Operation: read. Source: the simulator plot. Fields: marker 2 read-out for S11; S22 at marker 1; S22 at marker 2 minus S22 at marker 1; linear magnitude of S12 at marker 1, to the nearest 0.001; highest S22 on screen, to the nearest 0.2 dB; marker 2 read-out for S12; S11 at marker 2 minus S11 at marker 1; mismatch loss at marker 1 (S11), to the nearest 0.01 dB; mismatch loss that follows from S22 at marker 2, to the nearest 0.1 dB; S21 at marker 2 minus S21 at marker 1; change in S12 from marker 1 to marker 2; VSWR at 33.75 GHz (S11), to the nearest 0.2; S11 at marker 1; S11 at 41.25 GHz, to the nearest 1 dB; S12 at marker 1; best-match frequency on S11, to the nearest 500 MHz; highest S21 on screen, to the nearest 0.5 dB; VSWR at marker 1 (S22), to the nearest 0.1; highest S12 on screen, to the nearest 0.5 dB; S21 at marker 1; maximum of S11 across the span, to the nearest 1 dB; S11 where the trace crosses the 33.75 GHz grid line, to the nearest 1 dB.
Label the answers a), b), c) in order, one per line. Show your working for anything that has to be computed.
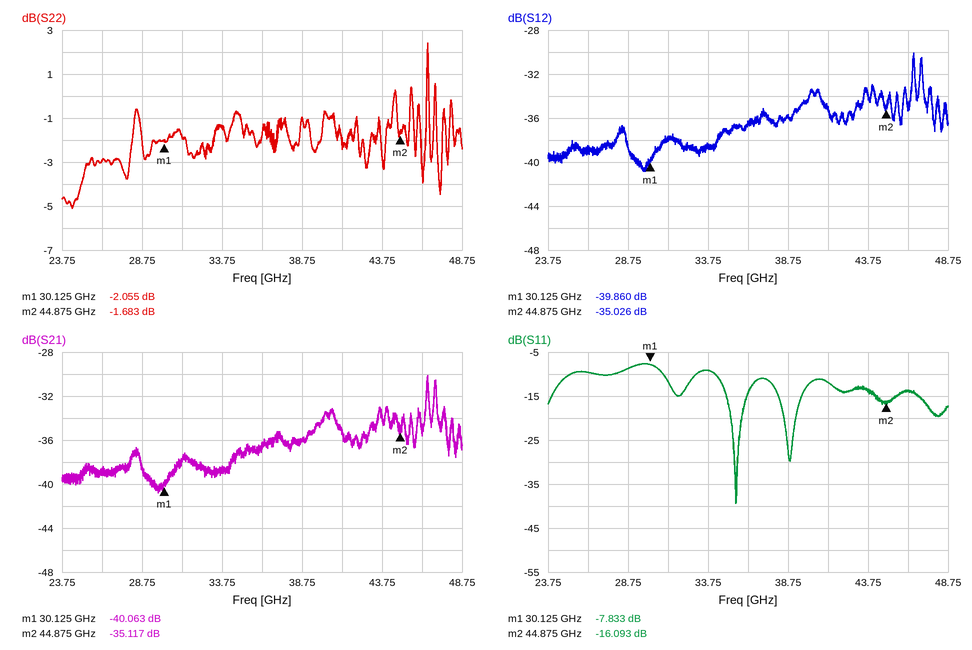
a) -16.093 dB
b) -2.055 dB
c) -1.683 − (-2.055) = 0.372 dB
d) 10^(-39.86/20) ≈ 0.010
e) 2.4 dB
f) -35.026 dB
g) -16.093 − (-7.833) = -8.260 dB
h) −10 log10(1 − 10^(-7.833/10)) ≈ 0.78 dB
i) −10 log10(1 − 10^(-1.683/10)) ≈ 4.9 dB
j) -35.117 − (-40.063) = 4.946 dB
k) -35.026 − (-39.86) = 4.834 dB
l) |Γ| = 10^(-9/20) = 0.3548; VSWR = (1 + 0.3548)/(1 − 0.3548) ≈ 2.10, so 2.0 to the nearest 0.2
m) -7.833 dB
n) -12 dB
o) -39.860 dB
p) 35.5 GHz
q) -30.0 dB
r) (1 + 0.7893)/(1 − 0.7893) ≈ 8.5
s) -30.0 dB
t) -40.063 dB
u) -8 dB
v) -9 dB
